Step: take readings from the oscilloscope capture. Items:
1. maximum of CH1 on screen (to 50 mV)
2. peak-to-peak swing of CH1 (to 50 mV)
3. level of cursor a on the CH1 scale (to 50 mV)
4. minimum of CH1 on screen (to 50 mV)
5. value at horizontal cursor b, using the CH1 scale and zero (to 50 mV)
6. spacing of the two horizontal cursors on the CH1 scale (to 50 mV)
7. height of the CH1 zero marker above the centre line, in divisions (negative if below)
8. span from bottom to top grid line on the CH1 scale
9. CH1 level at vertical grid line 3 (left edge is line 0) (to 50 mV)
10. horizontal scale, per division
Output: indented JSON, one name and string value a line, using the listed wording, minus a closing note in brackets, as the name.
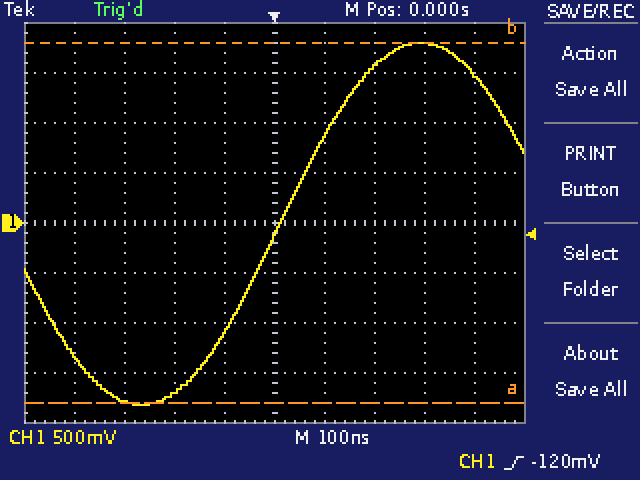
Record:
{
  "maximum of CH1 on screen": "1.80 V",
  "peak-to-peak swing of CH1": "3.60 V",
  "level of cursor a on the CH1 scale": "-1.80 V",
  "minimum of CH1 on screen": "-1.80 V",
  "value at horizontal cursor b, using the CH1 scale and zero": "1.80 V",
  "spacing of the two horizontal cursors on the CH1 scale": "3.60 V",
  "height of the CH1 zero marker above the centre line, in divisions": "0.0 div",
  "span from bottom to top grid line on the CH1 scale": "4 V",
  "CH1 level at vertical grid line 3 (left edge is line 0)": "-1.70 V",
  "horizontal scale, per division": "100 ns"
}
